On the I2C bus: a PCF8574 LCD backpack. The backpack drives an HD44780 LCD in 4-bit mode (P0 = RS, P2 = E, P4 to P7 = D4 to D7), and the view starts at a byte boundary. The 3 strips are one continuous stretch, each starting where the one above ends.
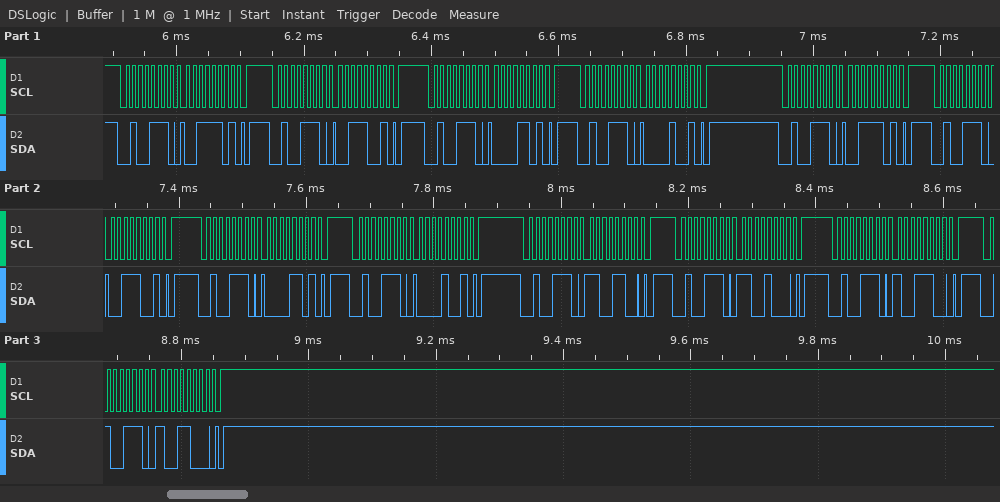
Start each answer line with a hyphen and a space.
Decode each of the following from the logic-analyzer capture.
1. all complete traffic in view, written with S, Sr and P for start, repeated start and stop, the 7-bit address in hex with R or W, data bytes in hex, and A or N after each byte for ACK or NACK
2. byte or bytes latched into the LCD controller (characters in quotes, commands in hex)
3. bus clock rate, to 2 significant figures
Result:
- S 27W A 3D A P S 27W A 39 A P S 27W A 0D A P S 27W A 09 A P S 27W A 3D A P S 27W A 39 A P S 27W A 0D A P S 27W A 09 A P S 27W A CC A P S 27W A C8 A P S 27W A 9C A P S 27W A 98 A P
- '0' '0' 0xC9
- 100 kHz
